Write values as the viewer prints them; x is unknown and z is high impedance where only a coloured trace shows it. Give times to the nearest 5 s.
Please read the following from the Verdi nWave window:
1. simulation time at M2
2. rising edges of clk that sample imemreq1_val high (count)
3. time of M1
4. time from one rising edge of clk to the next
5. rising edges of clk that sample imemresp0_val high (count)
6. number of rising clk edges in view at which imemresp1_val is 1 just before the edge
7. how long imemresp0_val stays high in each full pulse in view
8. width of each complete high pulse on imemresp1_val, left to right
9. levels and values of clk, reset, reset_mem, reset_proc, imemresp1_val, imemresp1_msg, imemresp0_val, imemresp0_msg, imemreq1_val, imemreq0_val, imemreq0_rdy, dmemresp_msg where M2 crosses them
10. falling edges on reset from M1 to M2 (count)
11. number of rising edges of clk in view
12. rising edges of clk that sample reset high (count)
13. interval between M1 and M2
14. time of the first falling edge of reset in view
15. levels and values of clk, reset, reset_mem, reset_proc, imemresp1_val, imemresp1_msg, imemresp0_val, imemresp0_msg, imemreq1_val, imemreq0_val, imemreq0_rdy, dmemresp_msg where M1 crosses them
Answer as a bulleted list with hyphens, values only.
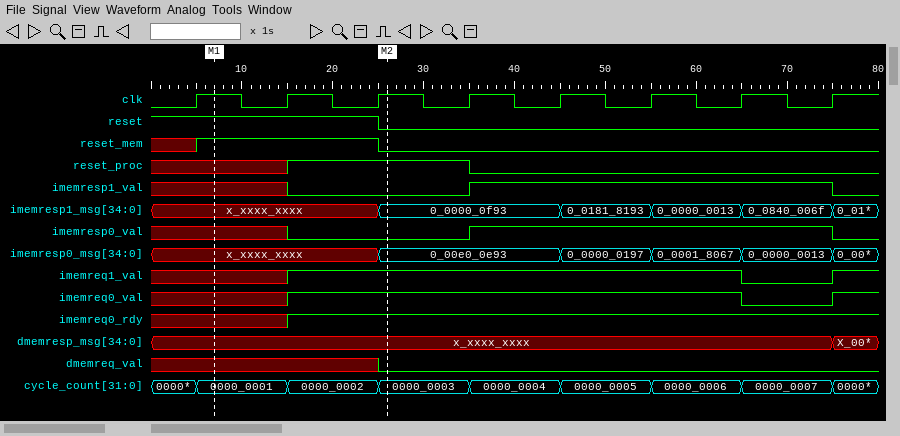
- 25 s
- 5
- 5 s
- 10 s
- 4
- 4
- 40 s
- 40 s
- clk=1, reset=0, reset_mem=0, reset_proc=1, imemresp1_val=0, imemresp1_msg=0_0000_0f93, imemresp0_val=0, imemresp0_msg=0_00e0_0e93, imemreq1_val=1, imemreq0_val=1, imemreq0_rdy=1, dmemresp_msg=x_xxxx_xxxx
- 1
- 8
- 3
- 20 s
- 25 s
- clk=1, reset=1, reset_mem=1, reset_proc=x, imemresp1_val=x, imemresp1_msg=x_xxxx_xxxx, imemresp0_val=x, imemresp0_msg=x_xxxx_xxxx, imemreq1_val=x, imemreq0_val=x, imemreq0_rdy=x, dmemresp_msg=x_xxxx_xxxx
